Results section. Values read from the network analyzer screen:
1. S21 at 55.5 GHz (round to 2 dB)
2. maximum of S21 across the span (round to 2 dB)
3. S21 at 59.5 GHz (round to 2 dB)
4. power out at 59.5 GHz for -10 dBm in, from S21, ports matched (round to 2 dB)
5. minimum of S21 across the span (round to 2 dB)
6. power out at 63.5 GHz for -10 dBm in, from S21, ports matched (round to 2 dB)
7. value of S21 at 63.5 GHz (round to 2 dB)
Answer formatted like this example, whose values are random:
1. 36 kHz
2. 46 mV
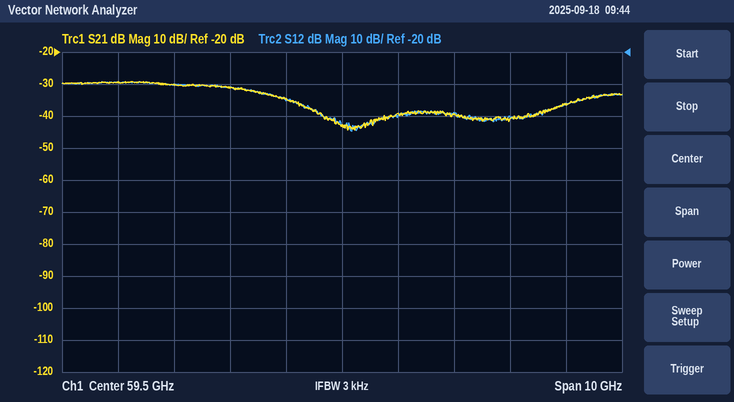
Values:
1. -30 dB
2. -30 dB
3. -42 dB
4. -52 dBm
5. -44 dB
6. -46 dBm
7. -36 dB
